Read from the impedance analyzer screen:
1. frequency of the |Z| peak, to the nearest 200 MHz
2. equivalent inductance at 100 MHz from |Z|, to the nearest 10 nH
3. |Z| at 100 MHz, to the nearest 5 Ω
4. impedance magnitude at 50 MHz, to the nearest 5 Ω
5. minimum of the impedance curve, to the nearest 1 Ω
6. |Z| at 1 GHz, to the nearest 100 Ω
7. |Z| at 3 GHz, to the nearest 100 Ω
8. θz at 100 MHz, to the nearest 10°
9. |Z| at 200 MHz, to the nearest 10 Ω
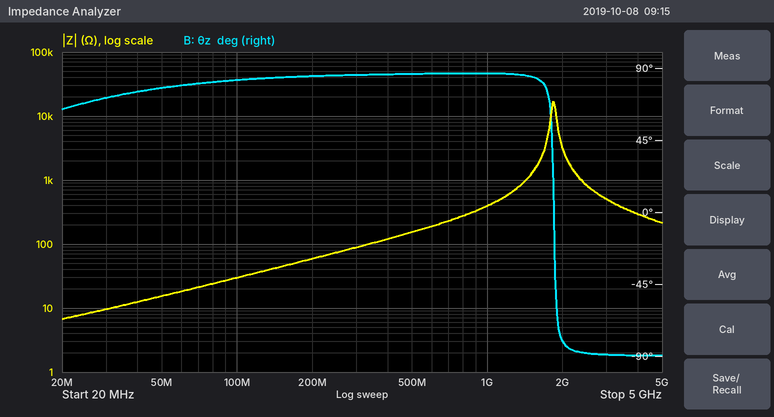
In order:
1.8 GHz
50 nH
30 Ω
15 Ω
7 Ω
400 Ω
500 Ω
80°
60 Ω
